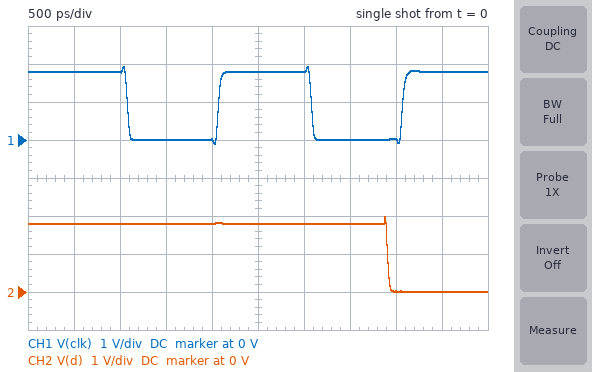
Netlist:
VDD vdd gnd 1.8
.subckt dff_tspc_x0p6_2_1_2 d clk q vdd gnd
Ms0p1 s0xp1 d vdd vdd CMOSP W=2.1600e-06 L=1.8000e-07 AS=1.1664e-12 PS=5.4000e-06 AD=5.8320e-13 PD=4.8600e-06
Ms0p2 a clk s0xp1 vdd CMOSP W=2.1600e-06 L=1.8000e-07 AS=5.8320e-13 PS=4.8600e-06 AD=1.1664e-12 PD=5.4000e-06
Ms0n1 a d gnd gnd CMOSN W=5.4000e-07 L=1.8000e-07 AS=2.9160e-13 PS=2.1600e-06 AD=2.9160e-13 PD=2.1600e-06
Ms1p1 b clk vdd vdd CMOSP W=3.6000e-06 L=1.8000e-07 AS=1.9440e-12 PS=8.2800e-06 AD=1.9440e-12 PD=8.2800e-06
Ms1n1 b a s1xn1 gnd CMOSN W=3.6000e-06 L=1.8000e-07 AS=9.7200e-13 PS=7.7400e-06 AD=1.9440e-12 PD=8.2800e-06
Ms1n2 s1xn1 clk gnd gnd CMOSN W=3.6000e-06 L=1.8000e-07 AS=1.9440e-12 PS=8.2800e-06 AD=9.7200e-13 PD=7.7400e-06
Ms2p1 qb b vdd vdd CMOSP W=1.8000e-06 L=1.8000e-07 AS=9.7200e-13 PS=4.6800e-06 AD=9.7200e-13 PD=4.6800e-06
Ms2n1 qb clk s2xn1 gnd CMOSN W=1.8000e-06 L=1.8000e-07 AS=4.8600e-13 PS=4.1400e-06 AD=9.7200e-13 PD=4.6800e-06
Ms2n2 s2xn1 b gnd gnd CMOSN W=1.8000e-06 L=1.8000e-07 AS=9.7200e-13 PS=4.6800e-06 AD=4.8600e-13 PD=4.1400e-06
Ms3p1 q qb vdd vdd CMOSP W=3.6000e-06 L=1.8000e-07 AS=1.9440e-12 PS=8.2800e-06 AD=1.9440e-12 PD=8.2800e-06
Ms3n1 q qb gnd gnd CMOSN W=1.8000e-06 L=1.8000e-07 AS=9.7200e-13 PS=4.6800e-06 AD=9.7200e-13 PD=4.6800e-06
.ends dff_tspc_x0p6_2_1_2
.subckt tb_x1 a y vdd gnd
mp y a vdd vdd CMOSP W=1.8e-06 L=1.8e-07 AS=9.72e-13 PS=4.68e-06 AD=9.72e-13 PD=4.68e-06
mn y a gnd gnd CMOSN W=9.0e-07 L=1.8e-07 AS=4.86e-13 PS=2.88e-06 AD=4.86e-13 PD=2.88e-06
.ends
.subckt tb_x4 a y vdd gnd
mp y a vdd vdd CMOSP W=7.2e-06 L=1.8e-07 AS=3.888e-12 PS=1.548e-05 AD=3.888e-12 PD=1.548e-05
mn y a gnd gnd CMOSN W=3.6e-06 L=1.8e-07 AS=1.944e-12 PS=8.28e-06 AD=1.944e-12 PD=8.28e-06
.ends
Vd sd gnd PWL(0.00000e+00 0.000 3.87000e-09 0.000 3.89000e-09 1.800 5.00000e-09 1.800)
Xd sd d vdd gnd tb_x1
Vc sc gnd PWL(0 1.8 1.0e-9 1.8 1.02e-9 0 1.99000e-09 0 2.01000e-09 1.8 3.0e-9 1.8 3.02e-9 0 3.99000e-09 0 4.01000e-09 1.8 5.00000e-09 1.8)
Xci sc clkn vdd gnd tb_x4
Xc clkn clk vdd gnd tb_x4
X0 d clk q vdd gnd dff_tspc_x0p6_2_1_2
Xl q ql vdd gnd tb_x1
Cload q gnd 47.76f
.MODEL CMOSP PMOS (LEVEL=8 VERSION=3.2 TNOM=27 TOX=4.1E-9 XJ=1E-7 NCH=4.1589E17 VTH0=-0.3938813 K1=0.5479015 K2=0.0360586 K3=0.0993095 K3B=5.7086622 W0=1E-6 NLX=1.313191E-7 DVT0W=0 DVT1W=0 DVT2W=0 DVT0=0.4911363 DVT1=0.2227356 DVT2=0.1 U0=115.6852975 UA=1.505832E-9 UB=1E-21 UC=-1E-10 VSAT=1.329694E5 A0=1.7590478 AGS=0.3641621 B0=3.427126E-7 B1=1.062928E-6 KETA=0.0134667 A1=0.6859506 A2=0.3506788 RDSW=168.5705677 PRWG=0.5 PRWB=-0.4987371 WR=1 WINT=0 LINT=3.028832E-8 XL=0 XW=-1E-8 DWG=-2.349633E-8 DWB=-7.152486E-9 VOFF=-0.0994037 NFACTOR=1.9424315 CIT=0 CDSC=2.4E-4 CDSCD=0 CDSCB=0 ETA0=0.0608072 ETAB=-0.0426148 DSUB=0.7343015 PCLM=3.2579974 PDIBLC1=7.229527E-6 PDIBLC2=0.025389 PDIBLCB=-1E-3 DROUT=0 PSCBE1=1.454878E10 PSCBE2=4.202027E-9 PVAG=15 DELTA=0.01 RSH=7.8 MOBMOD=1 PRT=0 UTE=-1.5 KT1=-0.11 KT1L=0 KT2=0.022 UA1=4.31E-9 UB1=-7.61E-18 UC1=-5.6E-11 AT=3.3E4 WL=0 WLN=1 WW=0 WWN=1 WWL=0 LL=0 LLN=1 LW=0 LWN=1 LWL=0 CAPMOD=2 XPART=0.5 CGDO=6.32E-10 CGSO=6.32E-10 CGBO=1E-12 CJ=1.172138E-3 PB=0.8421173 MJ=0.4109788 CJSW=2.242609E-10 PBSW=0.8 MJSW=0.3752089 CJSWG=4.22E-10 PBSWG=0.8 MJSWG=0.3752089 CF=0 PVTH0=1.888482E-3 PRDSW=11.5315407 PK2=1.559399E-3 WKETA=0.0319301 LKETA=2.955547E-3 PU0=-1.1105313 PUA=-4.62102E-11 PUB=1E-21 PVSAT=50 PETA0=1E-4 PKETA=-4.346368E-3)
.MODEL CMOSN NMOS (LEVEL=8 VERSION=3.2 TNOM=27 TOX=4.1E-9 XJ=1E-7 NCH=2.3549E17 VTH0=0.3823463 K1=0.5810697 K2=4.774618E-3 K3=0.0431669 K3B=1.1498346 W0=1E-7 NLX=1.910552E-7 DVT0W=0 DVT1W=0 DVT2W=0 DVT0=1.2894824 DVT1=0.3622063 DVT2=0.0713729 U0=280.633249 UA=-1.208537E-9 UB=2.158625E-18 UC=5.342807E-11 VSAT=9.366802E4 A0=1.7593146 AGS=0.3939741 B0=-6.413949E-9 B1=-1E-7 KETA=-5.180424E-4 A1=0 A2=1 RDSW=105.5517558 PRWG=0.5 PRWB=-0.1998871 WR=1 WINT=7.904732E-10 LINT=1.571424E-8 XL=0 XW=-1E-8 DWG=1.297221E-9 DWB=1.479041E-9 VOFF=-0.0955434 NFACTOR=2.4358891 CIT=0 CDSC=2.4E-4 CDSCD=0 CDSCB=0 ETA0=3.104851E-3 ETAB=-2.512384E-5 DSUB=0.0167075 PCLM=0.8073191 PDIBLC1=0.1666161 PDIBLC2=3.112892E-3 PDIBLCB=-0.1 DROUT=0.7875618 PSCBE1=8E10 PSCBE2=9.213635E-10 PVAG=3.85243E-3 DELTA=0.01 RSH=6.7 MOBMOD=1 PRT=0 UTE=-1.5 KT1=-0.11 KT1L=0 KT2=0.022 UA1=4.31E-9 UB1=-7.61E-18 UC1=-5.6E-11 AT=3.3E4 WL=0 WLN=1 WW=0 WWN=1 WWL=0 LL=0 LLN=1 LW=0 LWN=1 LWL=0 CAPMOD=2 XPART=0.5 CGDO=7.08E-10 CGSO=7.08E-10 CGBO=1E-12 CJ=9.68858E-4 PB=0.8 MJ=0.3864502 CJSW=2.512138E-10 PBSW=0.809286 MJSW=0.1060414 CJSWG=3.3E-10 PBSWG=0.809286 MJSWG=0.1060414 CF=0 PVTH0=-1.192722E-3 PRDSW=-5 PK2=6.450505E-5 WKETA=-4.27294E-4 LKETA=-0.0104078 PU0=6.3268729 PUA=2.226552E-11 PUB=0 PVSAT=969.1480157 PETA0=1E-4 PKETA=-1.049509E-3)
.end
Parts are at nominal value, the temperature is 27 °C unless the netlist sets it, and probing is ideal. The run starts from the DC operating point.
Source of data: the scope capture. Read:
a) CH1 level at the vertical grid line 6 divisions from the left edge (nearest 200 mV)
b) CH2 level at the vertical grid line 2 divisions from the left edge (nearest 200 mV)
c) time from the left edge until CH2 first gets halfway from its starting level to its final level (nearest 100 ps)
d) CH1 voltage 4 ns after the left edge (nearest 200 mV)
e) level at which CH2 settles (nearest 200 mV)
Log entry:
1.8 V
1.8 V
3.9 ns
0 V
0 V
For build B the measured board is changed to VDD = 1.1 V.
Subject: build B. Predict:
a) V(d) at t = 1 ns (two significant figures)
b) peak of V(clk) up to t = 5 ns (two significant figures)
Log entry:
1.1 V
1.2 V
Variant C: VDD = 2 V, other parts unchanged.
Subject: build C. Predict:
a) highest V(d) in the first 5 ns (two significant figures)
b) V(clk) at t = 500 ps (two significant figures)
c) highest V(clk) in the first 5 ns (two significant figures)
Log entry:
2.2 V
2.0 V
2.1 V
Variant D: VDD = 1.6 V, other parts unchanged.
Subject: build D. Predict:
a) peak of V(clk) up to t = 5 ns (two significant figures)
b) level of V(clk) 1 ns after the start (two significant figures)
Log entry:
1.7 V
1.6 V
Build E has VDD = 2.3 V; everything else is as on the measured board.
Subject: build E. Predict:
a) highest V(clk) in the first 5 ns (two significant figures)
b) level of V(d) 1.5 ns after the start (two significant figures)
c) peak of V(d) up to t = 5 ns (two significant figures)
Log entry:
2.4 V
2.3 V
2.5 V
